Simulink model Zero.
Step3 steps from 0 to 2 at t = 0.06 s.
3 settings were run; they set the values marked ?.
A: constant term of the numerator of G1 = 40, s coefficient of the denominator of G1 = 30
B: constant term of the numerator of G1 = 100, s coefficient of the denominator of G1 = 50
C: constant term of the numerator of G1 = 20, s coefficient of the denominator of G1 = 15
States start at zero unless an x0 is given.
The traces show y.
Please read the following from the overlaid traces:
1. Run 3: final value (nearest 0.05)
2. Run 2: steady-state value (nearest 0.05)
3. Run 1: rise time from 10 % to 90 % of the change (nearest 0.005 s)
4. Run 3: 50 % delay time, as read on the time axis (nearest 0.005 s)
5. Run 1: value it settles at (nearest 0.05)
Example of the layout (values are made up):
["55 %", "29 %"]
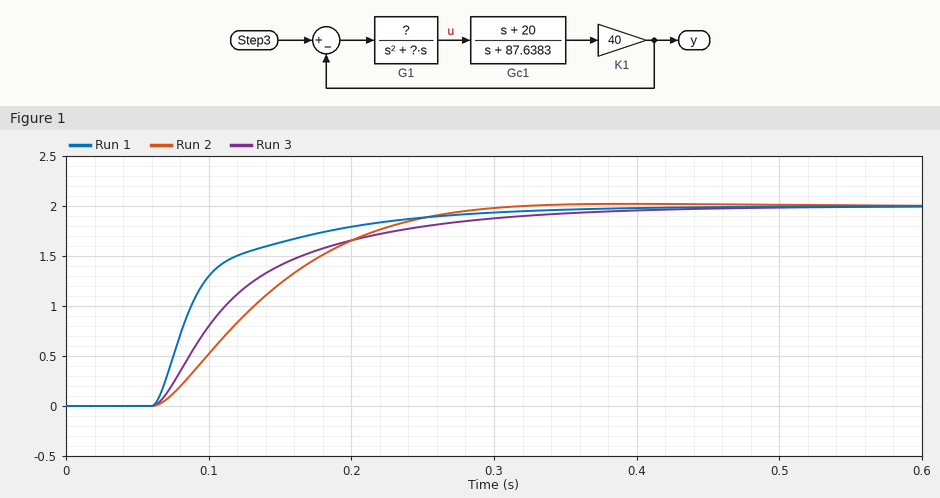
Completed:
["2.00", "2.00", "0.135 s", "0.110 s", "2.00"]
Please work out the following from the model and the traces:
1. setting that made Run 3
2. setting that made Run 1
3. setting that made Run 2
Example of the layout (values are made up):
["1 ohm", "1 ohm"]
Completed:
["A", "B", "C"]
